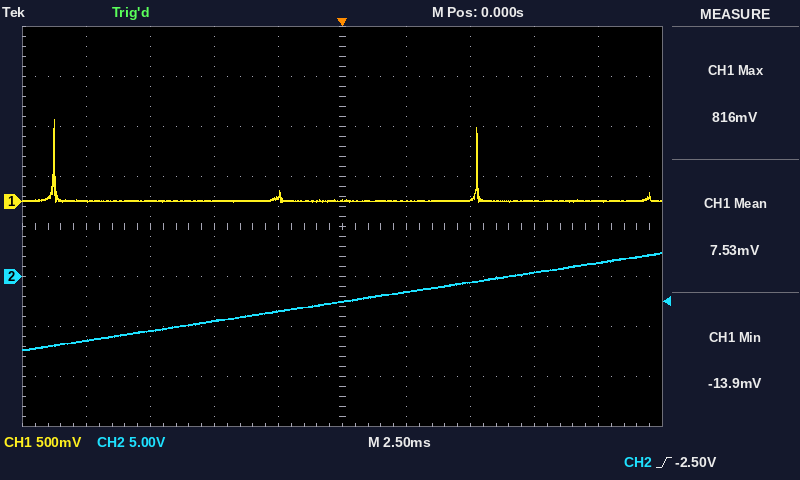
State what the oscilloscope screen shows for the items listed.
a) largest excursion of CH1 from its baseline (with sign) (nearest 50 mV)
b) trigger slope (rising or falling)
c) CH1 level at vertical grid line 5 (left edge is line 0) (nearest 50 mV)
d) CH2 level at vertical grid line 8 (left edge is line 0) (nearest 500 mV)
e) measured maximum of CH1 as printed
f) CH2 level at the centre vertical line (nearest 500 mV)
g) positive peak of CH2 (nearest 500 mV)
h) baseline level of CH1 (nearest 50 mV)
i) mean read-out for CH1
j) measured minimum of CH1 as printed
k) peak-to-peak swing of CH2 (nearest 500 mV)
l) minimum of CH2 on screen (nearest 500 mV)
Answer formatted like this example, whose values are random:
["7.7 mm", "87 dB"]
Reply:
["+800 mV", "rising", "0 mV", "500 mV", "816 mV", "-2.5 V", "2.5 V", "0 mV", "7.53 mV", "-13.9 mV", "10.0 V", "-7.5 V"]
